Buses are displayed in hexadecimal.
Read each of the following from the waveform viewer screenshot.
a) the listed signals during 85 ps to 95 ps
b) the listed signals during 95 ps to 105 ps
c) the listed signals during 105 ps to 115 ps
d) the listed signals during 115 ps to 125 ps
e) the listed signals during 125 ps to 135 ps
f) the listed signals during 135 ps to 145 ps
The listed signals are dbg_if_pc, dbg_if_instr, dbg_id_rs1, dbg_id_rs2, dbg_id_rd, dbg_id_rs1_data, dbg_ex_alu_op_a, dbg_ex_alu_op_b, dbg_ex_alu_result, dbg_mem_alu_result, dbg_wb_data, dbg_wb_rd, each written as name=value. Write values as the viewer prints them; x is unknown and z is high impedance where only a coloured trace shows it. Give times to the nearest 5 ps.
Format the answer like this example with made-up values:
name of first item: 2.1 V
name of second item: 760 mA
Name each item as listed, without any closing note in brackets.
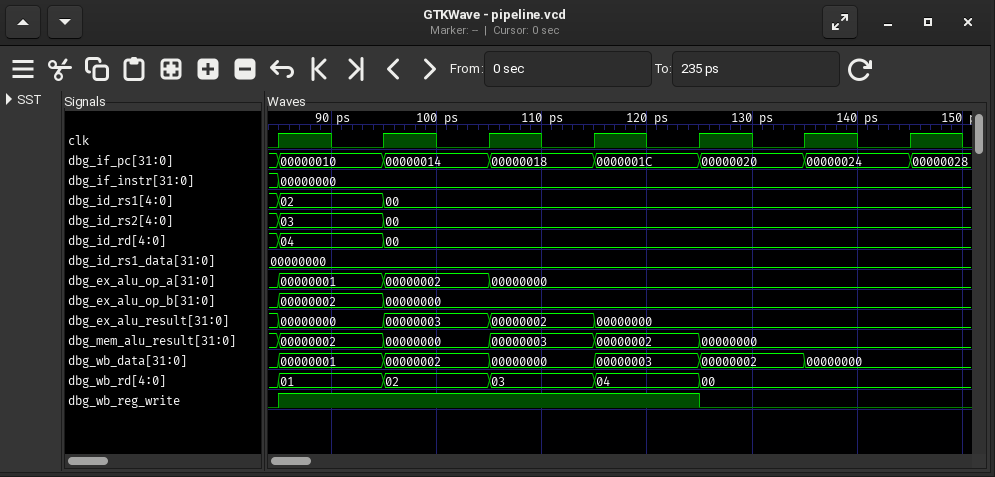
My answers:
the listed signals during 85 ps to 95 ps: dbg_if_pc=00000010, dbg_if_instr=00000000, dbg_id_rs1=02, dbg_id_rs2=03, dbg_id_rd=04, dbg_id_rs1_data=00000000, dbg_ex_alu_op_a=00000001, dbg_ex_alu_op_b=00000002, dbg_ex_alu_result=00000000, dbg_mem_alu_result=00000002, dbg_wb_data=00000001, dbg_wb_rd=01
the listed signals during 95 ps to 105 ps: dbg_if_pc=00000014, dbg_if_instr=00000000, dbg_id_rs1=00, dbg_id_rs2=00, dbg_id_rd=00, dbg_id_rs1_data=00000000, dbg_ex_alu_op_a=00000002, dbg_ex_alu_op_b=00000000, dbg_ex_alu_result=00000003, dbg_mem_alu_result=00000000, dbg_wb_data=00000002, dbg_wb_rd=02
the listed signals during 105 ps to 115 ps: dbg_if_pc=00000018, dbg_if_instr=00000000, dbg_id_rs1=00, dbg_id_rs2=00, dbg_id_rd=00, dbg_id_rs1_data=00000000, dbg_ex_alu_op_a=00000000, dbg_ex_alu_op_b=00000000, dbg_ex_alu_result=00000002, dbg_mem_alu_result=00000003, dbg_wb_data=00000000, dbg_wb_rd=03
the listed signals during 115 ps to 125 ps: dbg_if_pc=0000001C, dbg_if_instr=00000000, dbg_id_rs1=00, dbg_id_rs2=00, dbg_id_rd=00, dbg_id_rs1_data=00000000, dbg_ex_alu_op_a=00000000, dbg_ex_alu_op_b=00000000, dbg_ex_alu_result=00000000, dbg_mem_alu_result=00000002, dbg_wb_data=00000003, dbg_wb_rd=04
the listed signals during 125 ps to 135 ps: dbg_if_pc=00000020, dbg_if_instr=00000000, dbg_id_rs1=00, dbg_id_rs2=00, dbg_id_rd=00, dbg_id_rs1_data=00000000, dbg_ex_alu_op_a=00000000, dbg_ex_alu_op_b=00000000, dbg_ex_alu_result=00000000, dbg_mem_alu_result=00000000, dbg_wb_data=00000002, dbg_wb_rd=00
the listed signals during 135 ps to 145 ps: dbg_if_pc=00000024, dbg_if_instr=00000000, dbg_id_rs1=00, dbg_id_rs2=00, dbg_id_rd=00, dbg_id_rs1_data=00000000, dbg_ex_alu_op_a=00000000, dbg_ex_alu_op_b=00000000, dbg_ex_alu_result=00000000, dbg_mem_alu_result=00000000, dbg_wb_data=00000000, dbg_wb_rd=00
